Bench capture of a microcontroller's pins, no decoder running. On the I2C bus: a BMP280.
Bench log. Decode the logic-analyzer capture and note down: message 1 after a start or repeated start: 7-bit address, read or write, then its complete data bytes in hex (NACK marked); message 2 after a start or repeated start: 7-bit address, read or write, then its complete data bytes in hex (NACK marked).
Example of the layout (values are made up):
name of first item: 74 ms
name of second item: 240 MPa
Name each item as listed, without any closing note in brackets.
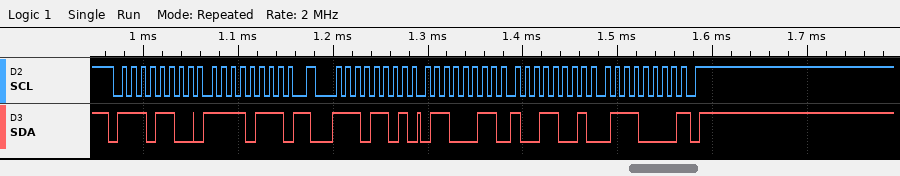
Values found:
message 1 after a start or repeated start: 7-bit address, read or write, then its complete data bytes in hex: 0x76 write: F7
message 2 after a start or repeated start: 7-bit address, read or write, then its complete data bytes in hex: 0x76 read: 63 99 70 NACK
